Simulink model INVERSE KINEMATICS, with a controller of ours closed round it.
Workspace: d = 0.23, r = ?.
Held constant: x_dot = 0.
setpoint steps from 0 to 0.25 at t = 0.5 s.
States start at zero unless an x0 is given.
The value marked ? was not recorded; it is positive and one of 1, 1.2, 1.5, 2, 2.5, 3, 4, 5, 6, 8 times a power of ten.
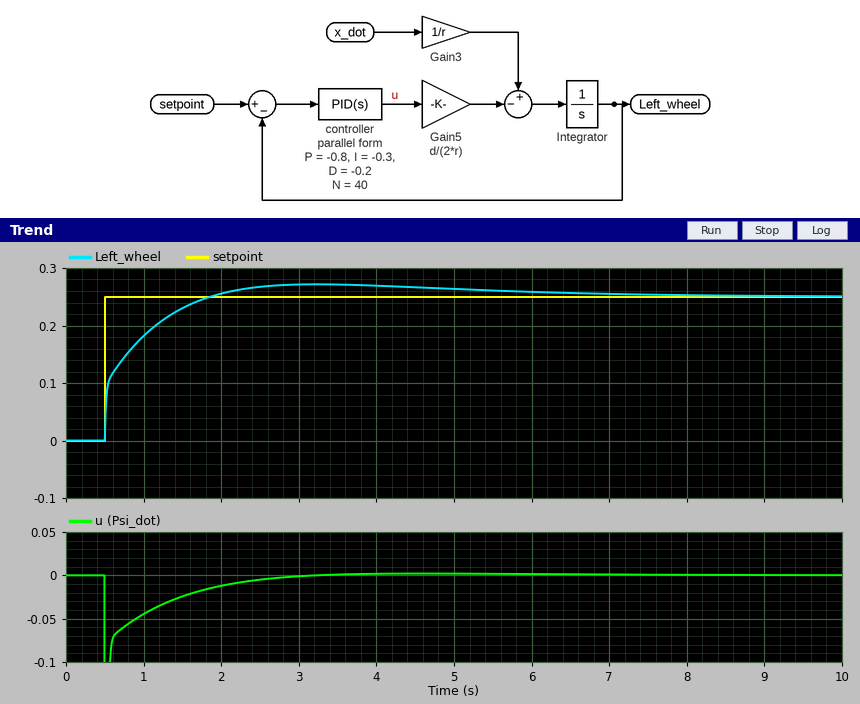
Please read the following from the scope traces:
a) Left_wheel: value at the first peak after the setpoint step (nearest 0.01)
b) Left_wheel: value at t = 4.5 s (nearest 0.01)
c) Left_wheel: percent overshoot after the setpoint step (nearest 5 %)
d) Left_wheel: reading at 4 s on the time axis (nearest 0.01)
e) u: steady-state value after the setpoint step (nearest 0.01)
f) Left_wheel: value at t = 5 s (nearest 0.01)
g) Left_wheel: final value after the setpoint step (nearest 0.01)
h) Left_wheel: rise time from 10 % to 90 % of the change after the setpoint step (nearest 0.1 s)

0.27
0.27
10 %
0.27
0.00
0.26
0.25
0.9 s
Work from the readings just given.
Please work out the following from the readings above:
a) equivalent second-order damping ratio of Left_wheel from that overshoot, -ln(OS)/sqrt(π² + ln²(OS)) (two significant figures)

0.59
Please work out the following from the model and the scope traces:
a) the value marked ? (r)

0.04
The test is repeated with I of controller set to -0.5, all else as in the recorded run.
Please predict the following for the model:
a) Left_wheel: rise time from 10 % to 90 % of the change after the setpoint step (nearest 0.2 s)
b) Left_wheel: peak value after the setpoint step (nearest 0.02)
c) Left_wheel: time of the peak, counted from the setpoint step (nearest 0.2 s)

0.8 s
0.28
2.2 s
